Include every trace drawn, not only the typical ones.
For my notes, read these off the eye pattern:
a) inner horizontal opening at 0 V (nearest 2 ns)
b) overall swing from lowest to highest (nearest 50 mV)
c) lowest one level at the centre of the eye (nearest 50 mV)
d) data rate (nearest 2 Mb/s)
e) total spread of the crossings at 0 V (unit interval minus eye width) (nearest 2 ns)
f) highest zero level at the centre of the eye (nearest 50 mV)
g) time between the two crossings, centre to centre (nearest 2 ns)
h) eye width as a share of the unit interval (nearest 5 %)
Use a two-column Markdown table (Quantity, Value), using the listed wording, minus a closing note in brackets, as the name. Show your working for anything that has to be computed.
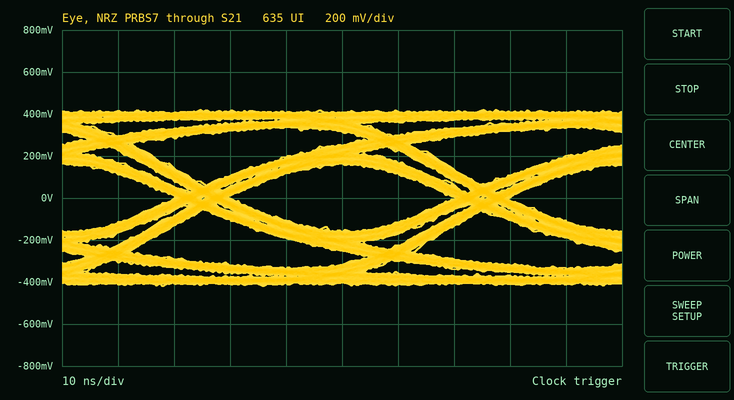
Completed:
| Quantity | Value |
|---|---|
| inner horizontal opening at 0 V | 40 ns |
| overall swing from lowest to highest | 850 mV |
| lowest one level at the centre of the eye | 150 mV |
| data rate | 20 Mb/s |
| total spread of the crossings at 0 V (unit interval minus eye width) | 10 ns |
| highest zero level at the centre of the eye | -150 mV |
| time between the two crossings, centre to centre | 50 ns |
| eye width as a share of the unit interval | 40 ns / 50 ns ≈ 80 % |
